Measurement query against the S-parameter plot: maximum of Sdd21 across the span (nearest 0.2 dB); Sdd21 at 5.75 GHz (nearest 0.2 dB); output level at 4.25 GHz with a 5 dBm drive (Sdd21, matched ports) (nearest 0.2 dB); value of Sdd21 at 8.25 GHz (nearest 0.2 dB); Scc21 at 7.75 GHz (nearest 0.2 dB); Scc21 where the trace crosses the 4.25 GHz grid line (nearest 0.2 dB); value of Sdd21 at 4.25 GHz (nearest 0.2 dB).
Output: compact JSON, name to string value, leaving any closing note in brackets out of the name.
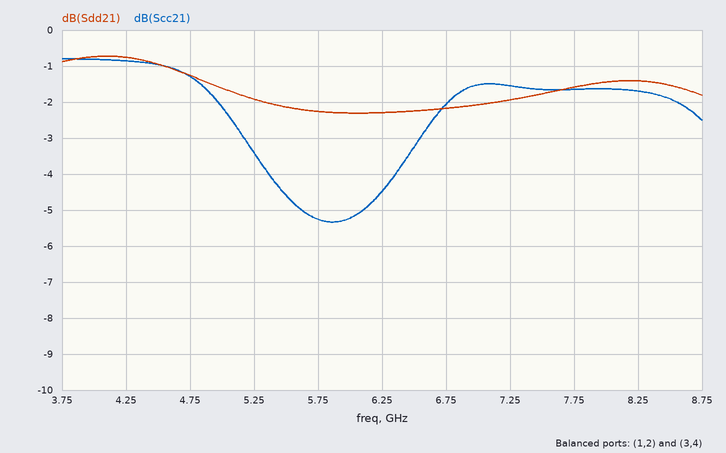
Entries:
{"maximum of Sdd21 across the span": "-0.8 dB", "Sdd21 at 5.75 GHz": "-2.2 dB", "output level at 4.25 GHz with a 5 dBm drive (Sdd21, matched ports)": "4.2 dBm", "value of Sdd21 at 8.25 GHz": "-1.4 dB", "Scc21 at 7.75 GHz": "-1.6 dB", "Scc21 where the trace crosses the 4.25 GHz grid line": "-0.8 dB", "value of Sdd21 at 4.25 GHz": "-0.8 dB"}
